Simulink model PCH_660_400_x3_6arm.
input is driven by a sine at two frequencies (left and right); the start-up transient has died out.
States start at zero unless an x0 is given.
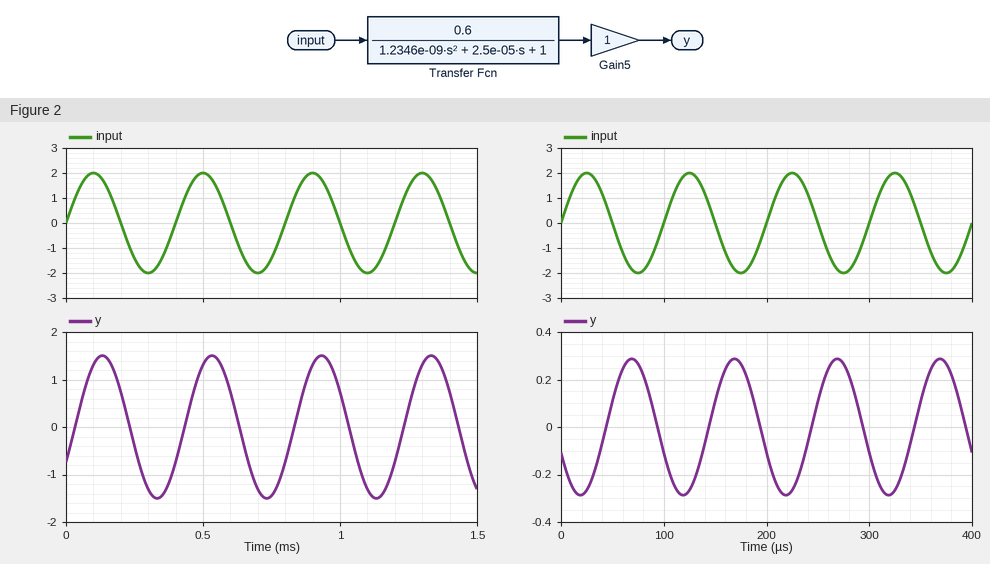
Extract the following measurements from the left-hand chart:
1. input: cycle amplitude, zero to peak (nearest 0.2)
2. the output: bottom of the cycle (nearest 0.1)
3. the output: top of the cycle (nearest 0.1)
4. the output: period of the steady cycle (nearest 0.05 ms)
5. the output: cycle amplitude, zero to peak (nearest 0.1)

2.0
-1.5
1.5
0.40 ms
1.5
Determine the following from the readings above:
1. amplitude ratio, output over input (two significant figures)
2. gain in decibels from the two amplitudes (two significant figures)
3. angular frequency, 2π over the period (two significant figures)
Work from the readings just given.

0.75
-2.5 dB
16 rad/ms
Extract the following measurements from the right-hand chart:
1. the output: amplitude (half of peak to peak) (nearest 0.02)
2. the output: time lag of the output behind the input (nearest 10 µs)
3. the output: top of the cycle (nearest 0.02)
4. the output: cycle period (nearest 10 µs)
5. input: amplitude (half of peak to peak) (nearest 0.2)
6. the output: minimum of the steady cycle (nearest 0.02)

0.28
40 µs
0.28
100 µs
2.0
-0.28
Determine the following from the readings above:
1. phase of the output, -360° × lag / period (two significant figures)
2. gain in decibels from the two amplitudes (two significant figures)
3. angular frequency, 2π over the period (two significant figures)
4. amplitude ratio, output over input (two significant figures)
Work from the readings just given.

-140°
-17 dB
0.063 rad/µs
0.14
